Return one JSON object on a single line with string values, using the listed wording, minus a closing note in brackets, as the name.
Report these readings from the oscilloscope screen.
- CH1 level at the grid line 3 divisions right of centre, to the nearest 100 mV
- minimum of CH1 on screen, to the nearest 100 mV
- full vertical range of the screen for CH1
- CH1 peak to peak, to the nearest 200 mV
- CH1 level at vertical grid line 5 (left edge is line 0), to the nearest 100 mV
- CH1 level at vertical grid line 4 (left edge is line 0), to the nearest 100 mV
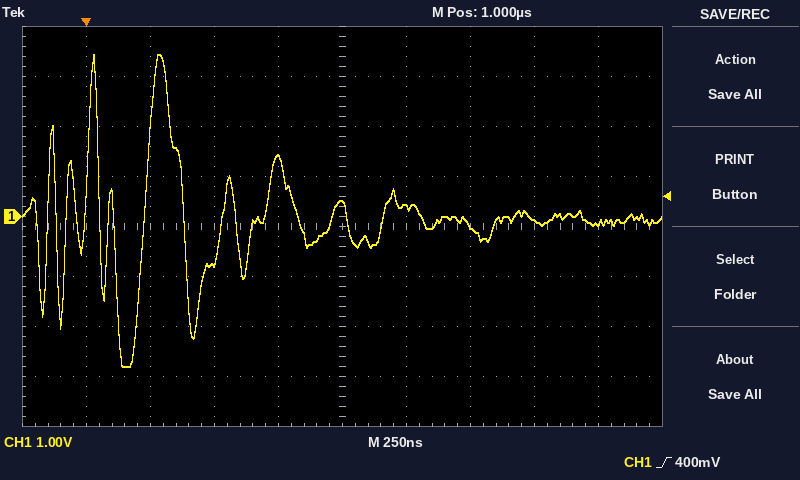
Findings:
{"CH1 level at the grid line 3 divisions right of centre, to the nearest 100 mV": "-100 mV", "minimum of CH1 on screen, to the nearest 100 mV": "-3.0 V", "full vertical range of the screen for CH1": "8 V", "CH1 peak to peak, to the nearest 200 mV": "6.2 V", "CH1 level at vertical grid line 5 (left edge is line 0), to the nearest 100 mV": "300 mV", "CH1 level at vertical grid line 4 (left edge is line 0), to the nearest 100 mV": "1.2 V"}
